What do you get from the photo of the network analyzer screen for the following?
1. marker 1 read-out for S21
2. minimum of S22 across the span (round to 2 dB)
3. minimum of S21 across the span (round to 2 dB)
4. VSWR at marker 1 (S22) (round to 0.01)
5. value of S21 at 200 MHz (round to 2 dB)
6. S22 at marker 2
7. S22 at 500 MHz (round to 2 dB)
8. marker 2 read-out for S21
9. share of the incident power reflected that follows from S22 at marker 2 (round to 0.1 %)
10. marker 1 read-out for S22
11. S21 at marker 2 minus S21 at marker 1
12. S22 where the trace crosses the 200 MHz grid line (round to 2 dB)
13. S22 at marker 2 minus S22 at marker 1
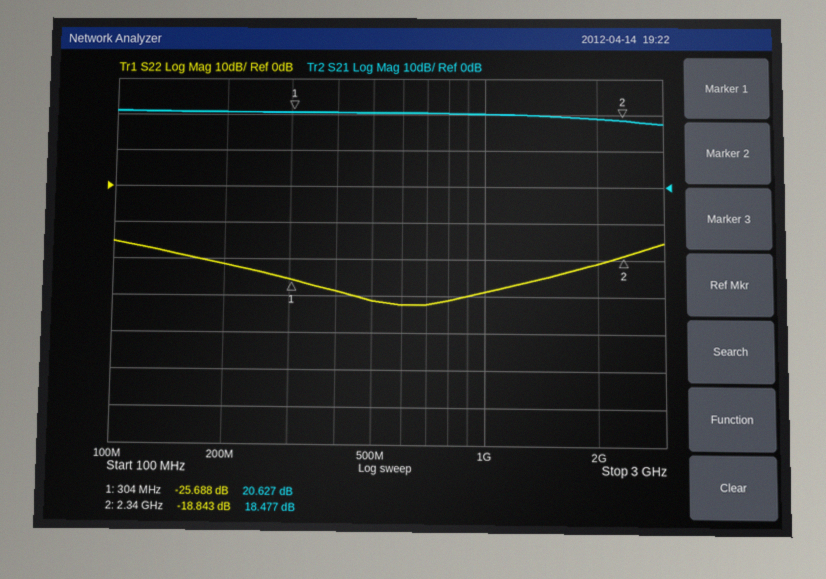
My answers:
20.627 dB
-32 dB
18 dB
1.11
20 dB
-18.843 dB
-32 dB
18.477 dB
1.3 %
-25.688 dB
-2.150 dB
-22 dB
6.845 dB
